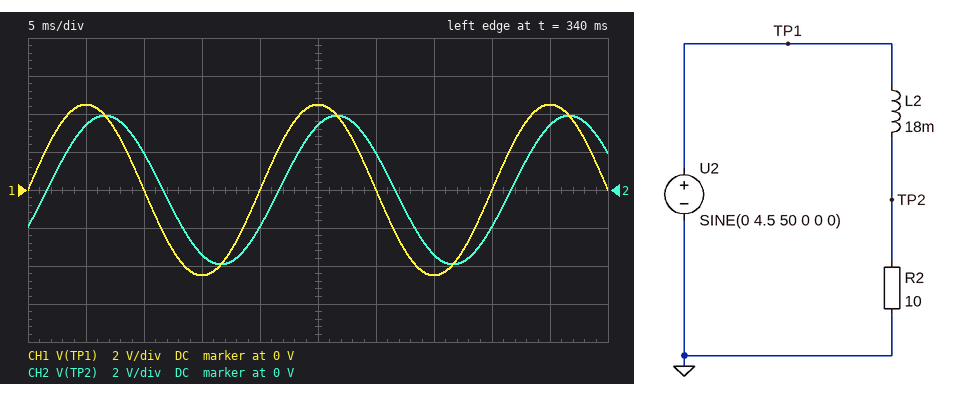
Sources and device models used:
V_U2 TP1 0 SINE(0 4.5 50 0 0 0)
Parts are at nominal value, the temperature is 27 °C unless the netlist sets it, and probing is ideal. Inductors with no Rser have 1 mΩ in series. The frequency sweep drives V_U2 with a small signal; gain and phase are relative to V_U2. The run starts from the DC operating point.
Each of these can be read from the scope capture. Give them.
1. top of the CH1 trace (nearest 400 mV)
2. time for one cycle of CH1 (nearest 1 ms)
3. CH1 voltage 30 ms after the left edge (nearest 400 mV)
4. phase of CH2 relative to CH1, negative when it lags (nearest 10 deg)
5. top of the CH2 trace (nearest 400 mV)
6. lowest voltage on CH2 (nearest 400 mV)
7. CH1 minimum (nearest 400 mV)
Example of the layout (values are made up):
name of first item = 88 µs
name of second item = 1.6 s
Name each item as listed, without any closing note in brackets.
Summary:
top of the CH1 trace = 4.4 V
time for one cycle of CH1 = 20 ms
CH1 voltage 30 ms after the left edge = 0 V
phase of CH2 relative to CH1, negative when it lags = -30 deg
top of the CH2 trace = 4.0 V
lowest voltage on CH2 = -4.0 V
CH1 minimum = -4.4 V
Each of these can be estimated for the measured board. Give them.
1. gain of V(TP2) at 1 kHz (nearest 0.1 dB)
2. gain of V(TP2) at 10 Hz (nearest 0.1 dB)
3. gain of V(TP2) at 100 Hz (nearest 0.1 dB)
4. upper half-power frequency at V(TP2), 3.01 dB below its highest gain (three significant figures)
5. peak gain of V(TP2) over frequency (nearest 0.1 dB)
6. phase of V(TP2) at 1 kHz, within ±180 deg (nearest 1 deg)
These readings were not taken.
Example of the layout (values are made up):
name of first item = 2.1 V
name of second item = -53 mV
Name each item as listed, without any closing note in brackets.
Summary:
gain of V(TP2) at 1 kHz = -21.1 dB
gain of V(TP2) at 10 Hz = -0.1 dB
gain of V(TP2) at 100 Hz = -3.6 dB
upper half-power frequency at V(TP2), 3.01 dB below its highest gain = 88.4 Hz
peak gain of V(TP2) over frequency = 0 dB
phase of V(TP2) at 1 kHz, within ±180 deg = -85 deg
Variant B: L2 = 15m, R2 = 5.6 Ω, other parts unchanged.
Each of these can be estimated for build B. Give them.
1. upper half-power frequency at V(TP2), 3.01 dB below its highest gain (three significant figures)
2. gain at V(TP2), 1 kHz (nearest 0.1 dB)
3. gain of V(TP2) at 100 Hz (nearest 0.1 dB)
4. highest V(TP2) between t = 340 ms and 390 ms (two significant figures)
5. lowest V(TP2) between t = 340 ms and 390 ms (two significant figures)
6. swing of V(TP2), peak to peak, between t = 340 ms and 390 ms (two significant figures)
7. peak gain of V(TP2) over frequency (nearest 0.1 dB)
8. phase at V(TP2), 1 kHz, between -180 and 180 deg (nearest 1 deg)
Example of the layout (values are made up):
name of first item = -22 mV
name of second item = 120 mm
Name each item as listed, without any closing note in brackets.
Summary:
upper half-power frequency at V(TP2), 3.01 dB below its highest gain = 59.4 Hz
gain at V(TP2), 1 kHz = -24.5 dB
gain of V(TP2) at 100 Hz = -5.8 dB
highest V(TP2) between t = 340 ms and 390 ms = 3.4 V
lowest V(TP2) between t = 340 ms and 390 ms = -3.4 V
swing of V(TP2), peak to peak, between t = 340 ms and 390 ms = 6.9 V
peak gain of V(TP2) over frequency = 0 dB
phase at V(TP2), 1 kHz, between -180 and 180 deg = -87 deg
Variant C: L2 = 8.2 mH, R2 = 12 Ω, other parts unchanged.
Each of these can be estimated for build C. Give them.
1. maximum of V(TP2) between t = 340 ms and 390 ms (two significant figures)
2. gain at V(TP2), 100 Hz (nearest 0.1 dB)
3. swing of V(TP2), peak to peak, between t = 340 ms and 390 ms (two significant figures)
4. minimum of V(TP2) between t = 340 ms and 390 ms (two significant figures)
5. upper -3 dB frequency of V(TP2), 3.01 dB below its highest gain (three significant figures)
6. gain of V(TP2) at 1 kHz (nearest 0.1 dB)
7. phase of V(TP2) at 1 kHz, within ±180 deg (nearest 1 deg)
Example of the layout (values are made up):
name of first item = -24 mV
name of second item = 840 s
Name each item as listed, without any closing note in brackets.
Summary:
maximum of V(TP2) between t = 340 ms and 390 ms = 4.4 V
gain at V(TP2), 100 Hz = -0.7 dB
swing of V(TP2), peak to peak, between t = 340 ms and 390 ms = 8.8 V
minimum of V(TP2) between t = 340 ms and 390 ms = -4.4 V
upper -3 dB frequency of V(TP2), 3.01 dB below its highest gain = 233 Hz
gain of V(TP2) at 1 kHz = -12.9 dB
phase of V(TP2) at 1 kHz, within ±180 deg = -77 deg
